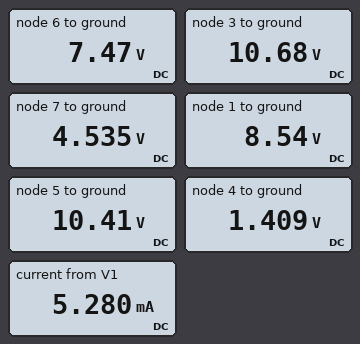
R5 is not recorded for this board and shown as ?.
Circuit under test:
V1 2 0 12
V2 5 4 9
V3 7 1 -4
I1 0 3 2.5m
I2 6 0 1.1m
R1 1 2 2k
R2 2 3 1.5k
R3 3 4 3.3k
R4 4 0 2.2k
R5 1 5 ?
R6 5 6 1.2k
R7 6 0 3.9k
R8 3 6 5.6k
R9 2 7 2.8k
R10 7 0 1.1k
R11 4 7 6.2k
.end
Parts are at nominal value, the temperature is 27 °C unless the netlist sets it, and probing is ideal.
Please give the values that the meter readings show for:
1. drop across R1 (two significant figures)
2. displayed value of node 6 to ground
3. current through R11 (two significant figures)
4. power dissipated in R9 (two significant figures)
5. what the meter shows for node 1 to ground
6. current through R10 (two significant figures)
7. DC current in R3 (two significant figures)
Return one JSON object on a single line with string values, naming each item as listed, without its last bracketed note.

{"drop across R1": "3.5 V", "displayed value of node 6 to ground": "7.47 V", "current through R11": "500 µA", "power dissipated in R9": "20 mW", "what the meter shows for node 1 to ground": "8.54 V", "current through R10": "4.1 mA", "DC current in R3": "2.8 mA"}
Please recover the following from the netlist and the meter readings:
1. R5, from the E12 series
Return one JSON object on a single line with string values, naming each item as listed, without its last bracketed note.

{"R5, from the E12 series": "8.2 kΩ"}
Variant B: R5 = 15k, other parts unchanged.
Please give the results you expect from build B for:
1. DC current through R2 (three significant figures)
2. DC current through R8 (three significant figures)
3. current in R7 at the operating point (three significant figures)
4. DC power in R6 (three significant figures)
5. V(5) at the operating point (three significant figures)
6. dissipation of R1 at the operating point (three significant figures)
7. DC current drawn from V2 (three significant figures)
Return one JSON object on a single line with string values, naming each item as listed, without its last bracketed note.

{"DC current through R2": "860 µA", "DC current through R8": "567 µA", "current in R7 at the operating point": "1.93 mA", "DC power in R6": "7.29 mW", "V(5) at the operating point": "10.5 V", "dissipation of R1 at the operating point": "6.15 mW", "DC current drawn from V2": "2.60 mA"}
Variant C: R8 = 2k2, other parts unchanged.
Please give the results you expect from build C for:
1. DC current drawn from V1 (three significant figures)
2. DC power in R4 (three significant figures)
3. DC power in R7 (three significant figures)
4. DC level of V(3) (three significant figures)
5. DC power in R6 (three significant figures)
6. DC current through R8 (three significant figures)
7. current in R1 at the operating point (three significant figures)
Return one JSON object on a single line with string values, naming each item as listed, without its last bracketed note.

{"DC current drawn from V1": "5.53 mA", "DC power in R4": "1.15 mW", "DC power in R7": "16.5 mW", "DC level of V(3)": "10.3 V", "DC power in R6": "5.48 mW", "DC current through R8": "1.02 mA", "current in R1 at the operating point": "1.72 mA"}
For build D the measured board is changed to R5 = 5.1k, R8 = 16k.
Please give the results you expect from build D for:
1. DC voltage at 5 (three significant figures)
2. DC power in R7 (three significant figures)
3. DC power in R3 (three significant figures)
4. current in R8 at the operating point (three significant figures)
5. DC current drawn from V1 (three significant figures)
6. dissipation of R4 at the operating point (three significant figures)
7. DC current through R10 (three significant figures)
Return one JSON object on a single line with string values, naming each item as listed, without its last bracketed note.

{"DC voltage at 5": "10.2 V", "DC power in R7": "12.6 mW", "DC power in R3": "28.9 mW", "current in R8 at the operating point": "246 µA", "DC current drawn from V1": "5.08 mA", "dissipation of R4 at the operating point": "634 µW", "DC current through R10": "4.15 mA"}
